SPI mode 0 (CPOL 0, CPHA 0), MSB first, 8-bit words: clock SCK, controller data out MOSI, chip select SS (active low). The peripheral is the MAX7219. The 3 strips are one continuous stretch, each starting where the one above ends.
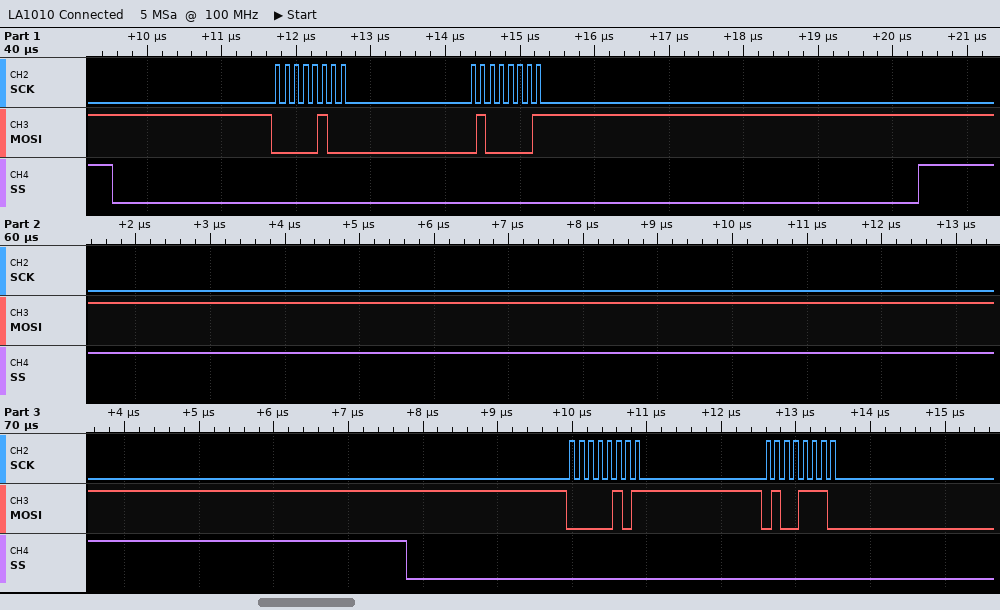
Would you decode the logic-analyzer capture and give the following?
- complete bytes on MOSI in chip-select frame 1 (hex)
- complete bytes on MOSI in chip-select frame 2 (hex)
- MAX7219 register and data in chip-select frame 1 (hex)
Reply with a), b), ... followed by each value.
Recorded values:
a) 04 41
b) 05 4E
c) register 0x4, data 0x41
